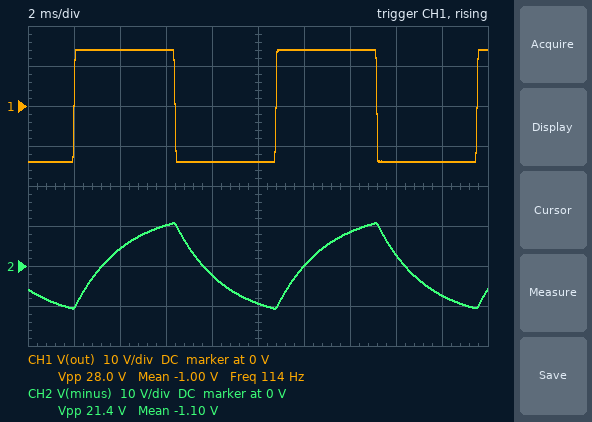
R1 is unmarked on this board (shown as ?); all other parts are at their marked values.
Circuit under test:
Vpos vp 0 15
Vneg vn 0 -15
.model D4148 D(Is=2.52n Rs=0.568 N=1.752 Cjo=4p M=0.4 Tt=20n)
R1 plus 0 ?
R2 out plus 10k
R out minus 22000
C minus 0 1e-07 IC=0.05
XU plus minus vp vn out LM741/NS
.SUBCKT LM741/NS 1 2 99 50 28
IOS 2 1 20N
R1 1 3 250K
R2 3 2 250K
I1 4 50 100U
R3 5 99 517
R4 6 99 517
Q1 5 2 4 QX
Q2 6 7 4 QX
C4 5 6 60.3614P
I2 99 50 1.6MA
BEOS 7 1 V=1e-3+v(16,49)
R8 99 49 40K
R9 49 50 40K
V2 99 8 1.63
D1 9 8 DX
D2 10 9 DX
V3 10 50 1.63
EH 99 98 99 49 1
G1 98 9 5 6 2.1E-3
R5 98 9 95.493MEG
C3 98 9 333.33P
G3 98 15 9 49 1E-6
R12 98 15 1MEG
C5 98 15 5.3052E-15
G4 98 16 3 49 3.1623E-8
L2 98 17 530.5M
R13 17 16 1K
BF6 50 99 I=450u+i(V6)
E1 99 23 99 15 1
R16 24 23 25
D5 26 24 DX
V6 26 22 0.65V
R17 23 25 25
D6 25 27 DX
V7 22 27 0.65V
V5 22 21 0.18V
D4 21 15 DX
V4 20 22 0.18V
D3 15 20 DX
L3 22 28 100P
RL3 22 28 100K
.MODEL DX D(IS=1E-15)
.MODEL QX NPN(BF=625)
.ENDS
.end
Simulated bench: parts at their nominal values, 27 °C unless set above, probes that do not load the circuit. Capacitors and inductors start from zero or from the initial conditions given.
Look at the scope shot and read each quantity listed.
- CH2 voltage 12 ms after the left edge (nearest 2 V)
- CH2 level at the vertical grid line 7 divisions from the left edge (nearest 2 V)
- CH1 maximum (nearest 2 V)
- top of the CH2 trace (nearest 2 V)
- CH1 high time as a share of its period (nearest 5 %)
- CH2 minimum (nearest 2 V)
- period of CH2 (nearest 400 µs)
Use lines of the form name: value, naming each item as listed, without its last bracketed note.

CH2 voltage 12 ms after the left edge: 0 V
CH2 level at the vertical grid line 7 divisions from the left edge: 8 V
CH1 maximum: 14 V
top of the CH2 trace: 10 V
CH1 high time as a share of its period: 50 %
CH2 minimum: -10 V
period of CH2: 8.8 ms
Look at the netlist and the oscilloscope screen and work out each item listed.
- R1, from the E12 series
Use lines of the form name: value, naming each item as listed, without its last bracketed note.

R1, from the E12 series: 33 kΩ
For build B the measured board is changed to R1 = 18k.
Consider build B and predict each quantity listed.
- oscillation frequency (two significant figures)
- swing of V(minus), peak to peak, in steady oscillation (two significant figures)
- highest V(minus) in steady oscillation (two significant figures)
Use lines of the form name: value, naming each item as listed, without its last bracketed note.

oscillation frequency: 150 Hz
swing of V(minus), peak to peak, in steady oscillation: 18 V
highest V(minus) in steady oscillation: 9.0 V
